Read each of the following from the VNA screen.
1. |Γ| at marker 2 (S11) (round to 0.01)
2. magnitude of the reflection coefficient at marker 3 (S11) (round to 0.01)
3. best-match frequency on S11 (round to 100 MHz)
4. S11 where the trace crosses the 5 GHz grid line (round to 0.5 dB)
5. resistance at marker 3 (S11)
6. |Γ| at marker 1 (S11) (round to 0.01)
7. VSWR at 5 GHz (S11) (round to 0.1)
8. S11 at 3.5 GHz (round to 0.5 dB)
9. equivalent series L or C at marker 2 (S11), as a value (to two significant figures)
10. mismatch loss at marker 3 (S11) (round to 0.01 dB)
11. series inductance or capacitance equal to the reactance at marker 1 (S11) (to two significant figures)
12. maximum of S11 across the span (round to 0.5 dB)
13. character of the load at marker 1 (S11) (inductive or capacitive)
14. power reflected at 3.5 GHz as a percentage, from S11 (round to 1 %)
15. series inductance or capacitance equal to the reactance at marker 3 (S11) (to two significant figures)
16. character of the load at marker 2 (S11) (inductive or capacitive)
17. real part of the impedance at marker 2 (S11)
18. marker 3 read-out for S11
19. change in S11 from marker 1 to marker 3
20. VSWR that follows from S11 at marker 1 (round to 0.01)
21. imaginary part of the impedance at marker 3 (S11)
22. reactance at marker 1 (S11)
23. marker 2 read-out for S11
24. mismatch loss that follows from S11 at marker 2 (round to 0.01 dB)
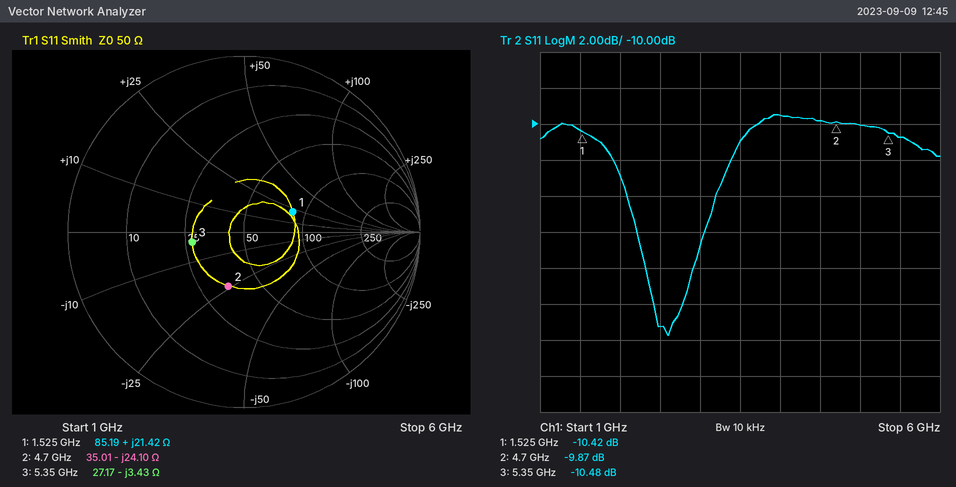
0.32
0.30
2.6 GHz
-10.0 dB
27.17 Ω
0.30
1.9
-11.0 dB
1.4 pF
0.41 dB
2.2 nH
-9.5 dB
inductive
8 %
8.7 pF
capacitive
35.01 Ω
-10.48 dB
-0.06 dB
1.86
-3.43 Ω
+21.42 Ω
-9.87 dB
0.47 dB
